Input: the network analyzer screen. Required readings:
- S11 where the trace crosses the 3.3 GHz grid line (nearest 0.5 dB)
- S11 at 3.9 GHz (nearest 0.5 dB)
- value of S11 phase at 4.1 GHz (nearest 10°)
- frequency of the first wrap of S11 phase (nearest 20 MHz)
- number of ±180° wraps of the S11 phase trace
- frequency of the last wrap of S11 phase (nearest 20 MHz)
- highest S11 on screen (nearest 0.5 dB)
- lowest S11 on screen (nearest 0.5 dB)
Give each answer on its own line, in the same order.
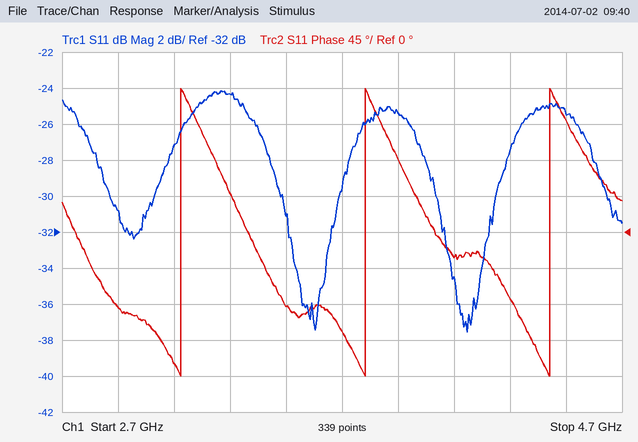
-24.5 dB
-25.5 dB
-30°
3.12 GHz
3
4.44 GHz
-24.0 dB
-37.5 dB
